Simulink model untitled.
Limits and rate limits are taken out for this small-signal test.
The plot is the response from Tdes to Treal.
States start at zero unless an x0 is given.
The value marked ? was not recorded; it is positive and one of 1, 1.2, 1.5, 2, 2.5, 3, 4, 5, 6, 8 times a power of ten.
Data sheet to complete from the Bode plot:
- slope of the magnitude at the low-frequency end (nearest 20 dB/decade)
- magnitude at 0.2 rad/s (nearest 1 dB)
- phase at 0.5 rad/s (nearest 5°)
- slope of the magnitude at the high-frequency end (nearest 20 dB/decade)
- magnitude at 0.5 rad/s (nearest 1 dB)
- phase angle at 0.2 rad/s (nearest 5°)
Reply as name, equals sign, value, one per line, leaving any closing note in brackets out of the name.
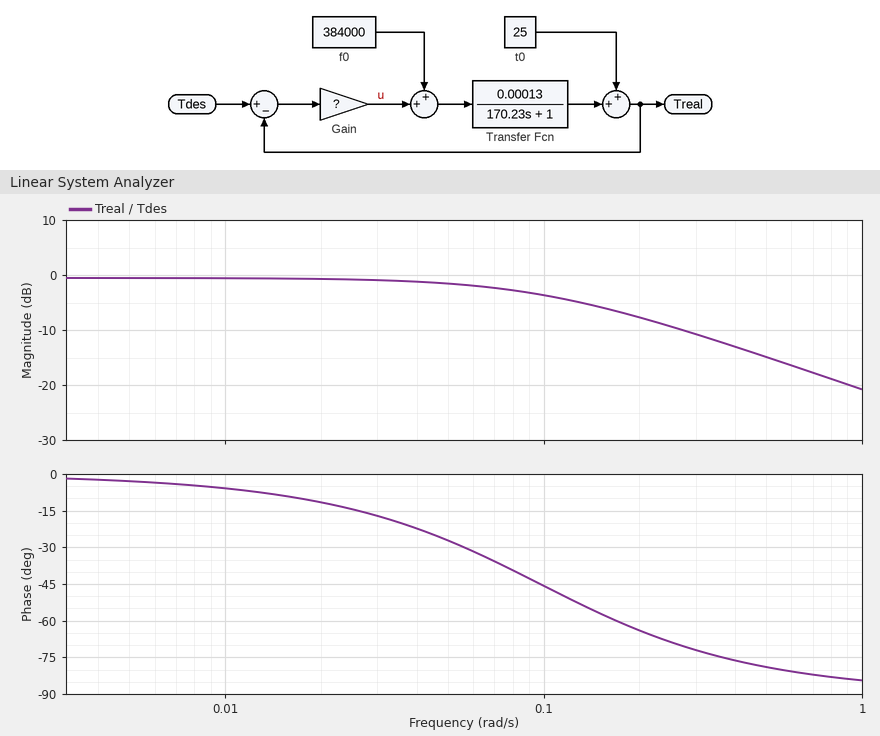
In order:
slope of the magnitude at the low-frequency end = 0 dB/decade
magnitude at 0.2 rad/s = -8 dB
phase at 0.5 rad/s = -80°
slope of the magnitude at the high-frequency end = -20 dB/decade
magnitude at 0.5 rad/s = -15 dB
phase angle at 0.2 rad/s = -65°
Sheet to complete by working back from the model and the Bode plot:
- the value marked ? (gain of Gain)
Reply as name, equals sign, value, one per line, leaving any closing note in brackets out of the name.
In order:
the value marked ? = 120000
